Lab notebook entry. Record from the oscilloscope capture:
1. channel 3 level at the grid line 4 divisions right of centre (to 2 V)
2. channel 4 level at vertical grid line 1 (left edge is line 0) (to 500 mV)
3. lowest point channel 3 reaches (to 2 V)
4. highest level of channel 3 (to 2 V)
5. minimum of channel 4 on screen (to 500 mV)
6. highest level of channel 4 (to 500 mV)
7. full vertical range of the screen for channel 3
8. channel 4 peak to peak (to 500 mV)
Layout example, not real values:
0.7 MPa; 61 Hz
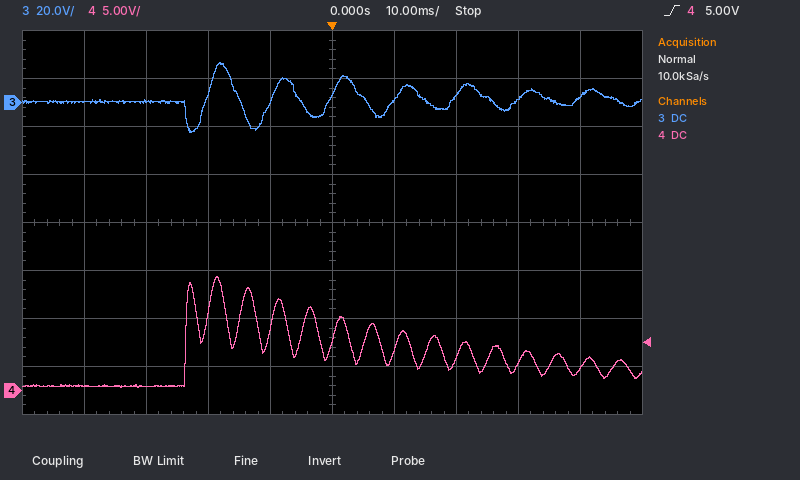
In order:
2 V; 500 mV; -12 V; 16 V; 500 mV; 12.0 V; 160 V; 11.5 V
